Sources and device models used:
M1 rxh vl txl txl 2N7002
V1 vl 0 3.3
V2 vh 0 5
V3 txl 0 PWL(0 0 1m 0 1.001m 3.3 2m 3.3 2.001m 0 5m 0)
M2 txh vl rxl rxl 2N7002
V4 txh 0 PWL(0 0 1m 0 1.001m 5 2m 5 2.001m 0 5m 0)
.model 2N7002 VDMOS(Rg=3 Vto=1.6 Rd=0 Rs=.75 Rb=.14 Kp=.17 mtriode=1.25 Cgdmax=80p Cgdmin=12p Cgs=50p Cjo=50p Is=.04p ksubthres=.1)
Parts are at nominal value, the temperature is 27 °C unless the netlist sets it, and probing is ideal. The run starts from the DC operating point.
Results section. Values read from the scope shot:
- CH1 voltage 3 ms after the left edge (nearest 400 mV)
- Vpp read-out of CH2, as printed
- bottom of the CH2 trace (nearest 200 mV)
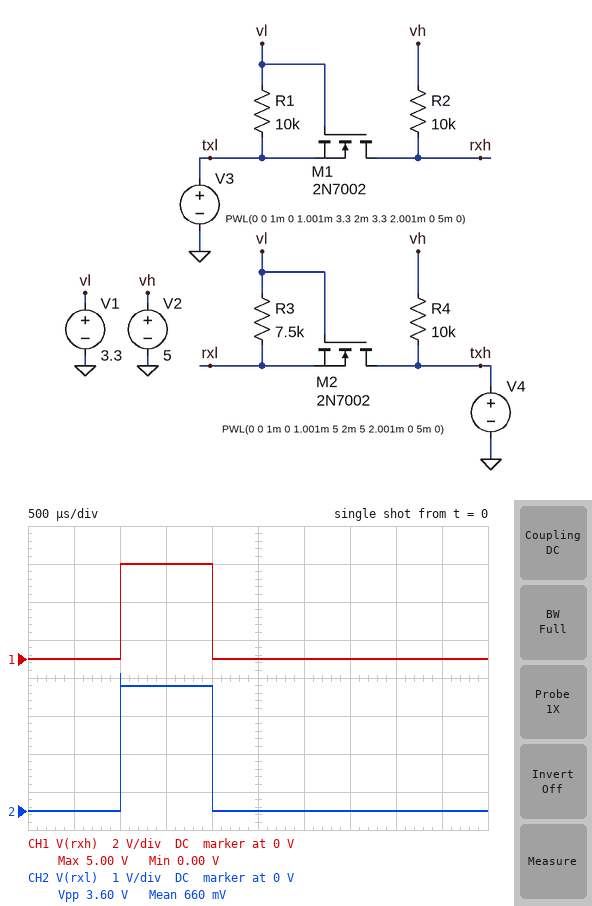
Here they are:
0 V
3.60 V
0 V
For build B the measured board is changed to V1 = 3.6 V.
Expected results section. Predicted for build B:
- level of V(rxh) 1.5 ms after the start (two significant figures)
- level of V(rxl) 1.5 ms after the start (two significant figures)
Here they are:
5.0 V
3.6 V
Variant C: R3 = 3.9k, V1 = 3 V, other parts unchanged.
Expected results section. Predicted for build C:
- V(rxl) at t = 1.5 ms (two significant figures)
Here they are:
3.0 V
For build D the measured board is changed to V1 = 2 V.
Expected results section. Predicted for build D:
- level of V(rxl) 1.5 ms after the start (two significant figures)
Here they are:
2.0 V
